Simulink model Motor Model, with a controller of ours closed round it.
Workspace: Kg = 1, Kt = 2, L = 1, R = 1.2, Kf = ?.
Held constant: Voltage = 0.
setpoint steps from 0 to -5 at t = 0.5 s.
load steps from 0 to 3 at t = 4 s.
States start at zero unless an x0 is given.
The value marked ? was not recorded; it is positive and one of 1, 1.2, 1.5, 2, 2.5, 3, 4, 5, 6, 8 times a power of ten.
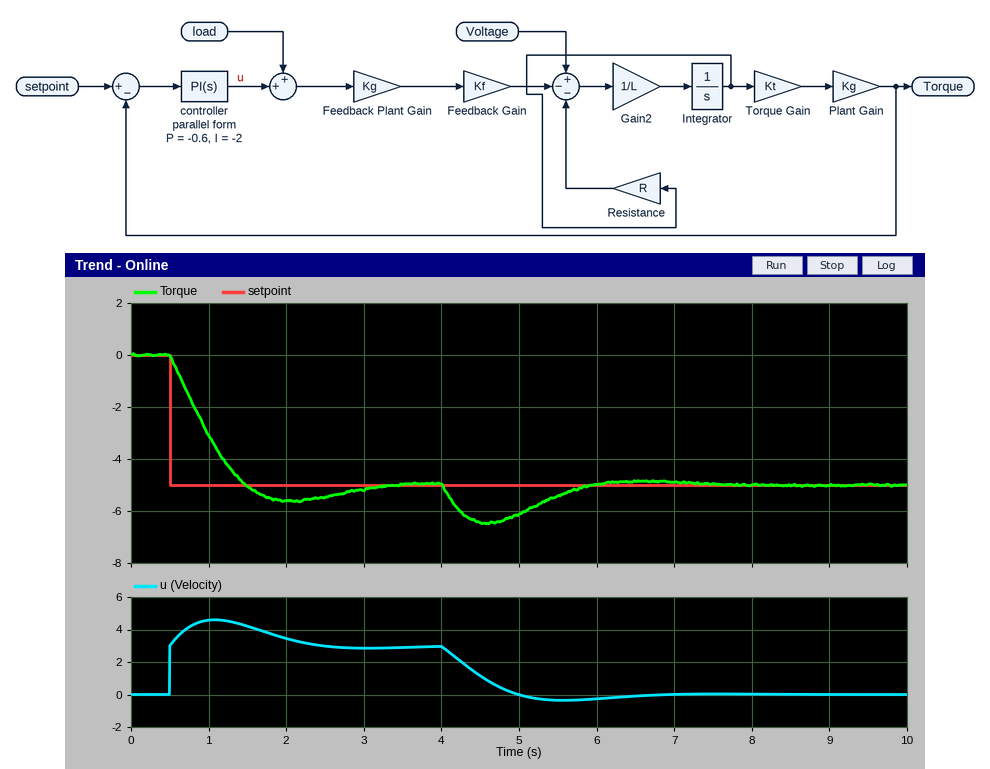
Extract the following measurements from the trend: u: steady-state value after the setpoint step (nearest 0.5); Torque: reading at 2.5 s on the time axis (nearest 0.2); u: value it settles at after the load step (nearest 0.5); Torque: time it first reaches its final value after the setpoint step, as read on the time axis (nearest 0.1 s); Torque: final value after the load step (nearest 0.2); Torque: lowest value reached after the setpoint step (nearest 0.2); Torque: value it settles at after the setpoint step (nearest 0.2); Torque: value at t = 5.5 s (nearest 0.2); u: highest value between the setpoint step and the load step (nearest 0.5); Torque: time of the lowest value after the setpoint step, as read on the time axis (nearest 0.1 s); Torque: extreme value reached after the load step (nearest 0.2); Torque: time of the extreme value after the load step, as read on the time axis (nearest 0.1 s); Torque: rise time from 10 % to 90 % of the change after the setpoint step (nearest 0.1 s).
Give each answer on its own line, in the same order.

3.0
-5.4
0.0
1.5 s
-5.0
-5.6
-5.0
-5.4
4.5
2.1 s
-6.4
4.6 s
0.7 s
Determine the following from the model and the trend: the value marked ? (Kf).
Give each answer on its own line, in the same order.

1
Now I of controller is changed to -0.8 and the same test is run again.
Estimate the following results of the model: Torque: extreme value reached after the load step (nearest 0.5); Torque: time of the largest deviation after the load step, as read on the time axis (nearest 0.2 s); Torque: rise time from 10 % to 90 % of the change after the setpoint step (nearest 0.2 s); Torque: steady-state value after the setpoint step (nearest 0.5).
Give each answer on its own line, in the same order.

-7.0
4.8 s
1.6 s
-5.0
